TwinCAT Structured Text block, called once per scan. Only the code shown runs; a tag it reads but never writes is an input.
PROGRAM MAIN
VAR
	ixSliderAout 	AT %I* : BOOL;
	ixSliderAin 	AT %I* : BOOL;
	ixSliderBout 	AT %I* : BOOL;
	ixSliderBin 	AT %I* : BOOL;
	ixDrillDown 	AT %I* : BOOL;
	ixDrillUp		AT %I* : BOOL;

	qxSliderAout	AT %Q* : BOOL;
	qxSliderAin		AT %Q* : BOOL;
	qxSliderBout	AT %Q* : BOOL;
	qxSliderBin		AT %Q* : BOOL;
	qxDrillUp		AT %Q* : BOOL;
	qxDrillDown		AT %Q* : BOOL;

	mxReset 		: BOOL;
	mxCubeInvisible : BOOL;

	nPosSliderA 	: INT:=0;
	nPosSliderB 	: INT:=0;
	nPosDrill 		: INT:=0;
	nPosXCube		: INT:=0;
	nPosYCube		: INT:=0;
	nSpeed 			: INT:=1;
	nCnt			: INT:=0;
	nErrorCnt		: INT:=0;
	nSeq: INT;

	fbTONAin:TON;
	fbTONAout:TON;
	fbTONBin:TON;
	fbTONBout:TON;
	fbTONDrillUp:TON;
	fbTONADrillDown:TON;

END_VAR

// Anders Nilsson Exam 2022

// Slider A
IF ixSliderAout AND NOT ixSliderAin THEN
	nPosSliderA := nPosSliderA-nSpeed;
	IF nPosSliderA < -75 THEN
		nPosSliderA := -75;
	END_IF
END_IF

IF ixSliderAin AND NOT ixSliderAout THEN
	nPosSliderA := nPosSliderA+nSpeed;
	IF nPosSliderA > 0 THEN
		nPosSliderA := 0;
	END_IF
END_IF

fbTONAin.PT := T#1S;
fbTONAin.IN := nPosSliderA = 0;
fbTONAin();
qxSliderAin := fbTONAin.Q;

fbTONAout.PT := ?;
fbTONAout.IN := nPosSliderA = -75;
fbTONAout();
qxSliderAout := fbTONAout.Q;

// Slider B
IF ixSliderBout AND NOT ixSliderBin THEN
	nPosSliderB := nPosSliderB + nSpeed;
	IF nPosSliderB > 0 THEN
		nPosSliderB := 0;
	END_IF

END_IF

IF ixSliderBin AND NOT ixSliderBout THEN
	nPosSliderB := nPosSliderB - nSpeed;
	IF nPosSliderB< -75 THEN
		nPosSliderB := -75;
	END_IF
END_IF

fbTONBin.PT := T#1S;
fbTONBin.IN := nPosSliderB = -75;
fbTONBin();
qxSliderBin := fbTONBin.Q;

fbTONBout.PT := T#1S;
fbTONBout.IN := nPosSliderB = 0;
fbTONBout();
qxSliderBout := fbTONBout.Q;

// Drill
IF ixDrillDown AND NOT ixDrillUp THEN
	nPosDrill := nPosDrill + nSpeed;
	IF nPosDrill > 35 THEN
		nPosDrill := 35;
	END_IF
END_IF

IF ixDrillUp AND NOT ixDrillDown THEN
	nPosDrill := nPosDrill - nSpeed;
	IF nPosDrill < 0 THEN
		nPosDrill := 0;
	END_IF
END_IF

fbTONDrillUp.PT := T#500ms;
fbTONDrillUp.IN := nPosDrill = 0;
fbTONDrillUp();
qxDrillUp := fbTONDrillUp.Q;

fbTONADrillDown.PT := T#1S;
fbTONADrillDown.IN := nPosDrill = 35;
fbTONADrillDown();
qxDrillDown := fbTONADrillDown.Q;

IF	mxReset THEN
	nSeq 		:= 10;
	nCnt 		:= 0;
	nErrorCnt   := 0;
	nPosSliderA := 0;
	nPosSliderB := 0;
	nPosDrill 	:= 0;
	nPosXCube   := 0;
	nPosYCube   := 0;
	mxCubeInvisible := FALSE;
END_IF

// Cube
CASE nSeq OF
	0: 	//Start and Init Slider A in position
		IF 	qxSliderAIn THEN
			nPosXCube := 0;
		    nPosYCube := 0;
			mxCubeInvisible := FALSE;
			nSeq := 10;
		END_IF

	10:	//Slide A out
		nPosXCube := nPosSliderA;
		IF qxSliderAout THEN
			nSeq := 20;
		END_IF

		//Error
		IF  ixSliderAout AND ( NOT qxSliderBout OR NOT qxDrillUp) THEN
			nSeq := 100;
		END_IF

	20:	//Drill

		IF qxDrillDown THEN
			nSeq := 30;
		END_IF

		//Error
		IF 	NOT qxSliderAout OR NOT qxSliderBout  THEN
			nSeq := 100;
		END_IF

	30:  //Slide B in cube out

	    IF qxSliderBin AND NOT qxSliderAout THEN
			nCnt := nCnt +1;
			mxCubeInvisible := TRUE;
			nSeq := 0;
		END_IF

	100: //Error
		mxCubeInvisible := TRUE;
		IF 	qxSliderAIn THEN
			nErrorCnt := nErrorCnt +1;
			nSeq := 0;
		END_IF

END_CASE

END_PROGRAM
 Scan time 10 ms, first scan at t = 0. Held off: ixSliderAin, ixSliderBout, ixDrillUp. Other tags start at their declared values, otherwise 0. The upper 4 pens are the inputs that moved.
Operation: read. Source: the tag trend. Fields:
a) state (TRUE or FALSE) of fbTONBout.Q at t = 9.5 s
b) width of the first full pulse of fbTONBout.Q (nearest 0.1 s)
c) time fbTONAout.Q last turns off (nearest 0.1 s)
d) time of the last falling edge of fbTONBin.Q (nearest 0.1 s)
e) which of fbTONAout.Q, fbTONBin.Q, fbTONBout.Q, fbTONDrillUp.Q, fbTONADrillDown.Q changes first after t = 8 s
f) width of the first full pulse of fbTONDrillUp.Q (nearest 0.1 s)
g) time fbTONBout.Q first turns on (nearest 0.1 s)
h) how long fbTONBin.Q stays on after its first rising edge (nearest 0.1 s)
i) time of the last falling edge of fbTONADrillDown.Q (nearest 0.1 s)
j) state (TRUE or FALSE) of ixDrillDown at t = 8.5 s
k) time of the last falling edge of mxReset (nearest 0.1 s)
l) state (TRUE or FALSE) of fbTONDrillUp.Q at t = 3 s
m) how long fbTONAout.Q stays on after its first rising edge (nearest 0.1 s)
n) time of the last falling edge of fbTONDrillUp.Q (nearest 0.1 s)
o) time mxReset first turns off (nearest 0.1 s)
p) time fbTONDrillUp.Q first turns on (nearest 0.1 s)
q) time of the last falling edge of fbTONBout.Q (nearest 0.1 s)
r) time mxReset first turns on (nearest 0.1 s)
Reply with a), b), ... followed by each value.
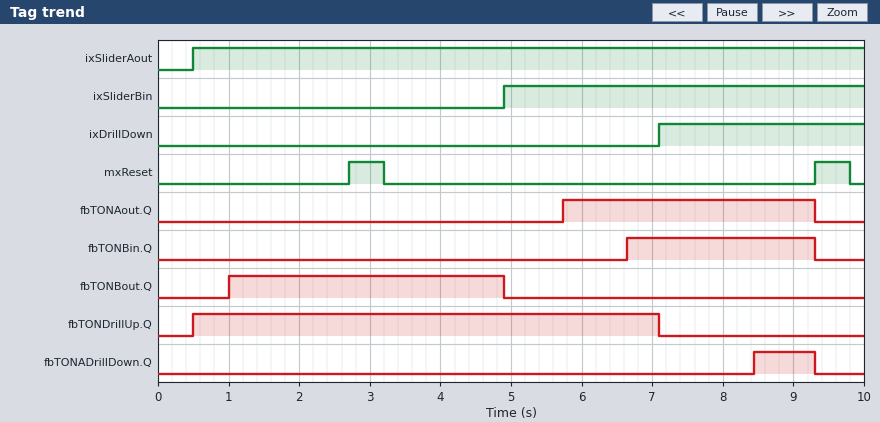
a) FALSE
b) 3.9 s
c) 9.3 s
d) 9.3 s
e) fbTONADrillDown.Q
f) 6.6 s
g) 1.0 s
h) 2.7 s
i) 9.3 s
j) TRUE
k) 9.8 s
l) TRUE
m) 3.6 s
n) 7.1 s
o) 3.2 s
p) 0.5 s
q) 4.9 s
r) 2.7 s
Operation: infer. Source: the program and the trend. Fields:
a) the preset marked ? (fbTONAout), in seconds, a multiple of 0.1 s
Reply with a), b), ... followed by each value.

a) 1.8 s
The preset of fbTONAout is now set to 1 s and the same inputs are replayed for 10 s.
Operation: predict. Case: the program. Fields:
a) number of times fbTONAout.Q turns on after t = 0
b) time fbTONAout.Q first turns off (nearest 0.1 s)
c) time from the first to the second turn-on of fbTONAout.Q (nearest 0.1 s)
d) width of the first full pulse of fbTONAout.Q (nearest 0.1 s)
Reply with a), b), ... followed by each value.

a) 2
b) 2.7 s
c) 2.7 s
d) 0.5 s
